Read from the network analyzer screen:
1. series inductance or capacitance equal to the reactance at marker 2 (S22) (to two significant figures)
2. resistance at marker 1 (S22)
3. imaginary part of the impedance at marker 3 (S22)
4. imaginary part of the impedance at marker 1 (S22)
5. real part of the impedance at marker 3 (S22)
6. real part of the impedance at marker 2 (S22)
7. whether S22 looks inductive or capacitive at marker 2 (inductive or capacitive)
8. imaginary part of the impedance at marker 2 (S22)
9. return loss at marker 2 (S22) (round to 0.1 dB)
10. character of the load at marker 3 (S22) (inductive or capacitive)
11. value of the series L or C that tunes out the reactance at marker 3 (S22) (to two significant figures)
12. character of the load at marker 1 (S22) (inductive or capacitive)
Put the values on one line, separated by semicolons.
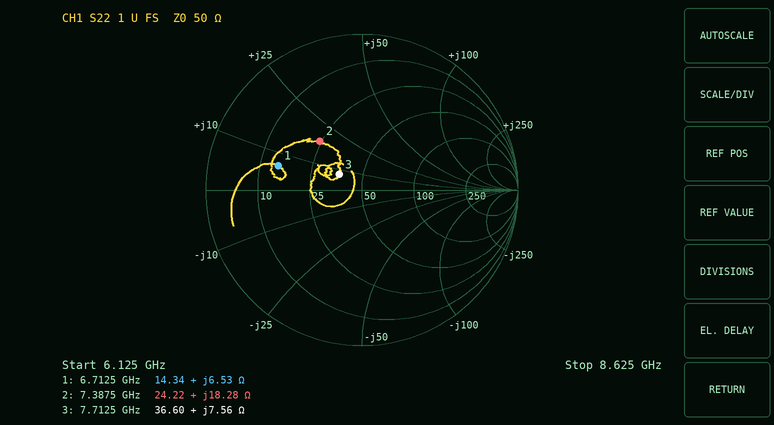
390 pH; 14.34 Ω; +7.56 Ω; +6.53 Ω; 36.60 Ω; 24.22 Ω; inductive; +18.28 Ω; 7.7 dB; inductive; 2.7 pF; inductive
